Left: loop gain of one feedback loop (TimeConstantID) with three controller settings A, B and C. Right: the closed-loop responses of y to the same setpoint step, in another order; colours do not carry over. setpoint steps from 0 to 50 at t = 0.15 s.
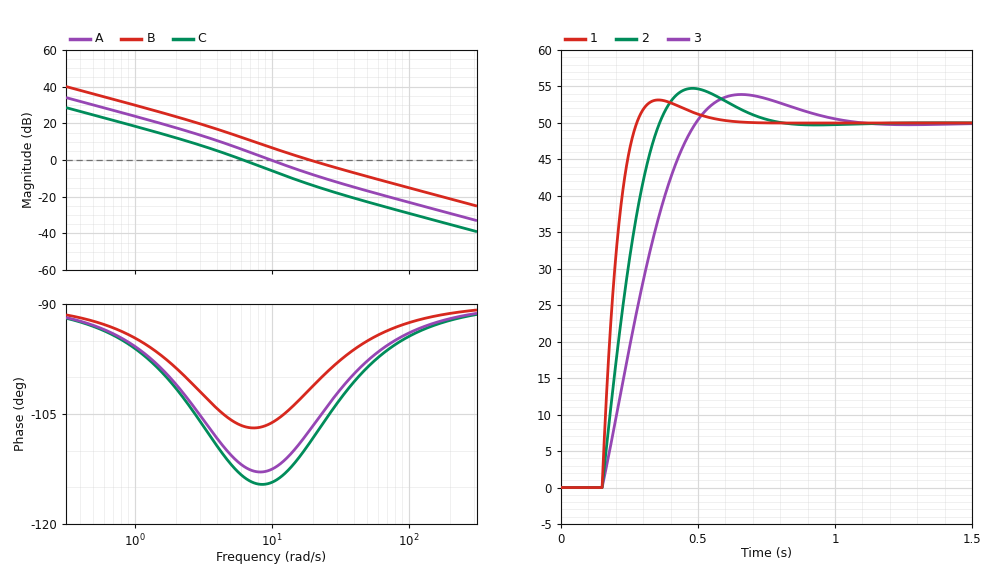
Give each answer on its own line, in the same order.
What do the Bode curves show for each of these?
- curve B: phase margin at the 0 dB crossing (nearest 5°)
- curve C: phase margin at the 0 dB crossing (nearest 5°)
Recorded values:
80°
65°
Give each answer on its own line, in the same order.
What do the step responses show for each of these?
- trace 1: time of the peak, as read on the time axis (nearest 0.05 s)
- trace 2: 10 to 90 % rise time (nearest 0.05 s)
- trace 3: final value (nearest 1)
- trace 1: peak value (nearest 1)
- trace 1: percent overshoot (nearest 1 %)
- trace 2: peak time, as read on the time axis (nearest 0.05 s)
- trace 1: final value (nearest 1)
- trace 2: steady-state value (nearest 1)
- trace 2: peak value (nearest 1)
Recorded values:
0.35 s
0.15 s
50
53
6 %
0.50 s
50
50
55
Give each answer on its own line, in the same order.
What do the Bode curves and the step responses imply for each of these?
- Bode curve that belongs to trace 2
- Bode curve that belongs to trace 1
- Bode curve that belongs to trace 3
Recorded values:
A
B
C
